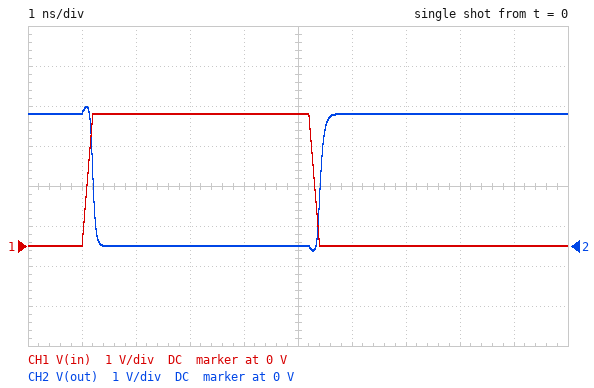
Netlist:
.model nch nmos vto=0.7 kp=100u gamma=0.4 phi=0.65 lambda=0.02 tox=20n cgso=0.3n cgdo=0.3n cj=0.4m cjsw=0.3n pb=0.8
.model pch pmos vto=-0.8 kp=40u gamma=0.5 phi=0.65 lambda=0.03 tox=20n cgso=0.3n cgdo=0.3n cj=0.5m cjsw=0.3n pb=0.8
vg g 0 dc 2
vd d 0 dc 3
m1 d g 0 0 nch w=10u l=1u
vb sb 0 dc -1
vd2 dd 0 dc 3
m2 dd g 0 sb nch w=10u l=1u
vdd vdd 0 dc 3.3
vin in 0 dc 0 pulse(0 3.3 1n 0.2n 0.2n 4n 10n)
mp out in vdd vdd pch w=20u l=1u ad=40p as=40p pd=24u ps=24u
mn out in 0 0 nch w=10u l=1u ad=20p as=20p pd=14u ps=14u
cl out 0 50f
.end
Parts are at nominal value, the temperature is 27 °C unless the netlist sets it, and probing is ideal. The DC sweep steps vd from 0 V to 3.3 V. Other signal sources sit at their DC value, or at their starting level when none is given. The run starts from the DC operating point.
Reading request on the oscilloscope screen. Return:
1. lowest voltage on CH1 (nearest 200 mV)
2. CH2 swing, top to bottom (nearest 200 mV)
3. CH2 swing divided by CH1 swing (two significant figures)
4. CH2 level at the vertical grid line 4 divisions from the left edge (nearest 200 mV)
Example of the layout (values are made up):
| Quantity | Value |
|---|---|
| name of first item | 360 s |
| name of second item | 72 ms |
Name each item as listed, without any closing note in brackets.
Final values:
| Quantity | Value |
|---|---|
| lowest voltage on CH1 | 0 V |
| CH2 swing, top to bottom | 3.6 V |
| CH2 swing divided by CH1 swing | 1.1 |
| CH2 level at the vertical grid line 4 divisions from the left edge | 0 V |
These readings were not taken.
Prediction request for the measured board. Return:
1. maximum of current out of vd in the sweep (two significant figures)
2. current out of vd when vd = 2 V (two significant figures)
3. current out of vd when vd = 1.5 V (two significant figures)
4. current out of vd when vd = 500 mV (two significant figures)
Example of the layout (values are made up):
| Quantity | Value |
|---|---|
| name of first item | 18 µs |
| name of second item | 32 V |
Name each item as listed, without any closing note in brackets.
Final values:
| Quantity | Value |
|---|---|
| maximum of current out of vd in the sweep | 900 µA |
| current out of vd when vd = 2 V | 880 µA |
| current out of vd when vd = 1.5 V | 870 µA |
| current out of vd when vd = 500 mV | 530 µA |
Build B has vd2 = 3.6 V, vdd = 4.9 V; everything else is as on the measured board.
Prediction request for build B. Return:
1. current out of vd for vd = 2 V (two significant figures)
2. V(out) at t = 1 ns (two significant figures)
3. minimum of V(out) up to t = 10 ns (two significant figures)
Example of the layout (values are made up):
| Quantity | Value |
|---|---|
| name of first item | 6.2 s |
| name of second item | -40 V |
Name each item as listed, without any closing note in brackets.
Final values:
| Quantity | Value |
|---|---|
| current out of vd for vd = 2 V | 880 µA |
| V(out) at t = 1 ns | 4.9 V |
| minimum of V(out) up to t = 10 ns | 92 mV |
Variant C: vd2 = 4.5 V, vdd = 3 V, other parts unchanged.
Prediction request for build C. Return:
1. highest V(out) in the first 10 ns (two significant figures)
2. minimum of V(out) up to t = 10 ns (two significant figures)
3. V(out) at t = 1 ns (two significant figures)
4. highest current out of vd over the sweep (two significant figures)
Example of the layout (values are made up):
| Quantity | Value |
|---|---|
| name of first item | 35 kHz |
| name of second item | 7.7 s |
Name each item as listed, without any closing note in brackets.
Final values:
| Quantity | Value |
|---|---|
| highest V(out) in the first 10 ns | 3.2 V |
| minimum of V(out) up to t = 10 ns | -140 mV |
| V(out) at t = 1 ns | 3.0 V |
| highest current out of vd over the sweep | 900 µA |
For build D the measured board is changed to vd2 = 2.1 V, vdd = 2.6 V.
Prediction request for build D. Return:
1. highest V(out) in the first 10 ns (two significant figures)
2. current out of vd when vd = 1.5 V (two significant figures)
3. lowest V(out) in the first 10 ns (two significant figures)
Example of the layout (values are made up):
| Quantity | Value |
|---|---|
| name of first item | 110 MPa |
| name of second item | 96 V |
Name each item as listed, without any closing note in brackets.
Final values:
| Quantity | Value |
|---|---|
| highest V(out) in the first 10 ns | 2.8 V |
| current out of vd when vd = 1.5 V | 870 µA |
| lowest V(out) in the first 10 ns | -180 mV |
